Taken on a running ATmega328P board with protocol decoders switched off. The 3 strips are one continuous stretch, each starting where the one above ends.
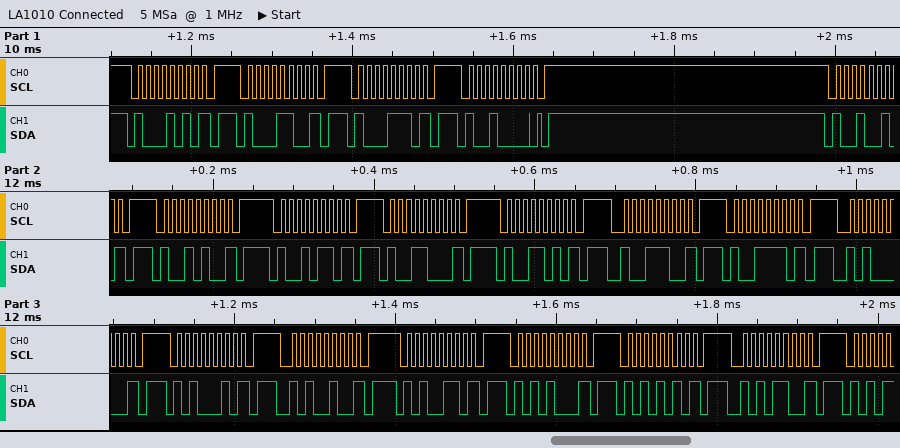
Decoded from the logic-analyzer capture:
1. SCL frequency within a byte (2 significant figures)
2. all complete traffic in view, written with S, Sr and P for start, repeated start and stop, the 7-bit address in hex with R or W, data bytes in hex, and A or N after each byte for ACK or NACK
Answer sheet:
100 kHz
S 45W N P S 46W N P S 47W N P S 48W A P S 49W N P S 4AW N P S 4BW N P S 4CW N P S 4DW N P S 4EW N P S 4FW N P S 50W N P S 51W N P S 52W N P S 53W N P S 54W N P S 55W N P S 56W N P
